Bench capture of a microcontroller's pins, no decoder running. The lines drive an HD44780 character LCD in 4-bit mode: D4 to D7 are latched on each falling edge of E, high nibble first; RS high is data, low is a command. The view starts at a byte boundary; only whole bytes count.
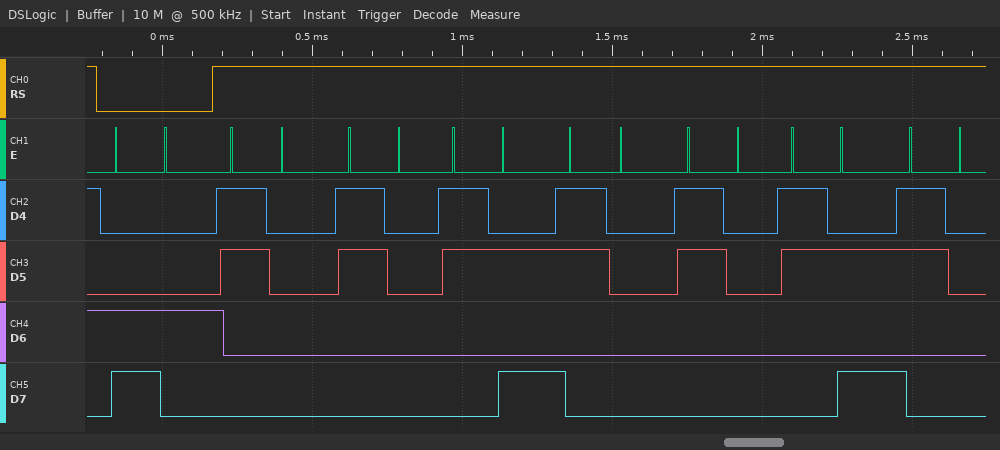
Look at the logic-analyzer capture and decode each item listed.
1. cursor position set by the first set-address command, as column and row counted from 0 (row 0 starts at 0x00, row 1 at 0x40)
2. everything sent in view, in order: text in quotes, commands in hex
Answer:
column 4, row 1
0xC4 "00:00:0"
